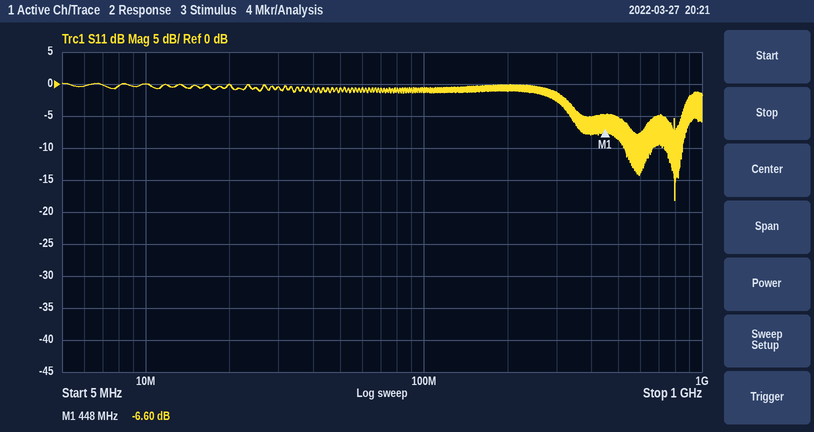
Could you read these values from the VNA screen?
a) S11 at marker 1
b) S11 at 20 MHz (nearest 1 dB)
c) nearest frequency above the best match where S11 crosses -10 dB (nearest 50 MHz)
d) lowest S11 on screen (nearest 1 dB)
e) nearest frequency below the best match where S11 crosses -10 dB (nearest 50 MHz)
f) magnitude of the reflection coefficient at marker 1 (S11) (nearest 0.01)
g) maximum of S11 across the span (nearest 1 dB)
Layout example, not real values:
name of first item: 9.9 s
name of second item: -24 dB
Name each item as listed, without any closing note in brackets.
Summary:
S11 at marker 1: -6.60 dB
S11 at 20 MHz: 0 dB
nearest frequency above the best match where S11 crosses -10 dB: 800 MHz
lowest S11 on screen: -18 dB
nearest frequency below the best match where S11 crosses -10 dB: 800 MHz
magnitude of the reflection coefficient at marker 1 (S11): 0.47
maximum of S11 across the span: 0 dB
